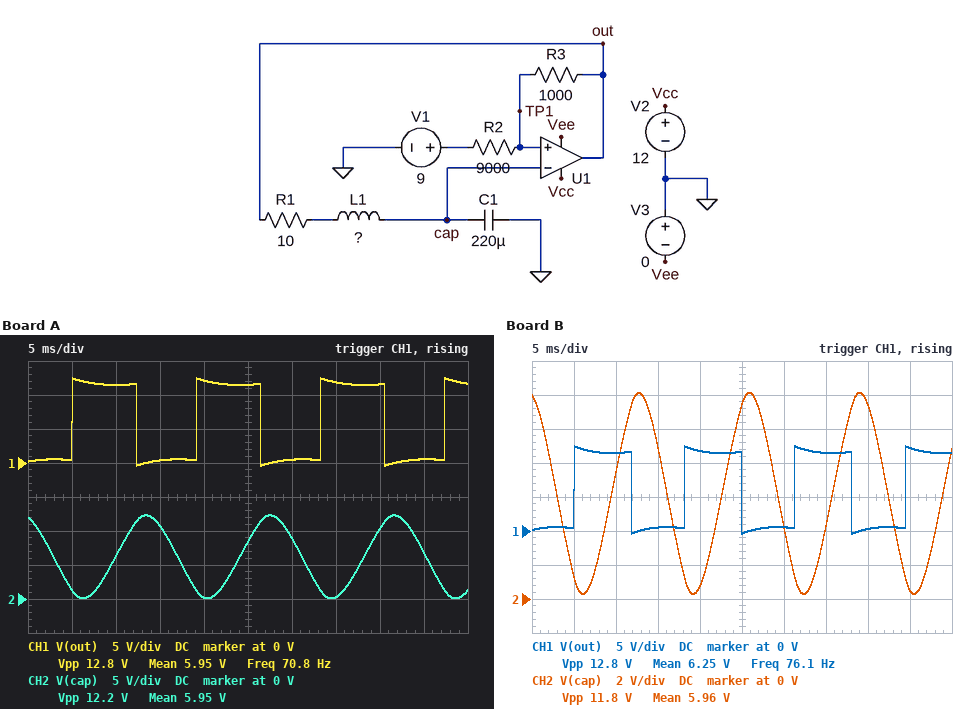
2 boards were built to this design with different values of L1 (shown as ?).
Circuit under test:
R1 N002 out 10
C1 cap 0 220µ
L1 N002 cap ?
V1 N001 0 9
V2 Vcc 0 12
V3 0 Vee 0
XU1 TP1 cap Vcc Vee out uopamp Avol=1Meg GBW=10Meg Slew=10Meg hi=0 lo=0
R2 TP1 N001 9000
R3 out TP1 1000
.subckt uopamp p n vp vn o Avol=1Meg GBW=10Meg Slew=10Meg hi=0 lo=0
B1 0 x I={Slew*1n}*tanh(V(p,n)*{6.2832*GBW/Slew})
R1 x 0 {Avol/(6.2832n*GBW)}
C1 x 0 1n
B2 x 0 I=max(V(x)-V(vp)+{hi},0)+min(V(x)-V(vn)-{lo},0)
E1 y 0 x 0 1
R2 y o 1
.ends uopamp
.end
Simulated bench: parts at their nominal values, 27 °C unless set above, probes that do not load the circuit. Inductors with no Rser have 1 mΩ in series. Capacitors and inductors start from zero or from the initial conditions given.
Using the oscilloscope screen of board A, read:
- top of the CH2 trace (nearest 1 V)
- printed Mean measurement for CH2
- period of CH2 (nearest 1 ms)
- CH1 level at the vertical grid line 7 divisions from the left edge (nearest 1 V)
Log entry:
12 V
5.95 V
14 ms
12 V
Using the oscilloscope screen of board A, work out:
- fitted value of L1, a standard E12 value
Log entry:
39 mH
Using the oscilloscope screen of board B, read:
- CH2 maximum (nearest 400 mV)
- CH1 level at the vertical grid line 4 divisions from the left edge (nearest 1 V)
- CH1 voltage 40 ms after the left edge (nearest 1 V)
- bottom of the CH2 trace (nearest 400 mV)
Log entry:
12.0 V
12 V
0 V
400 mV
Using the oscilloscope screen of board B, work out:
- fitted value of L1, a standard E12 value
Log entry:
33 mH
